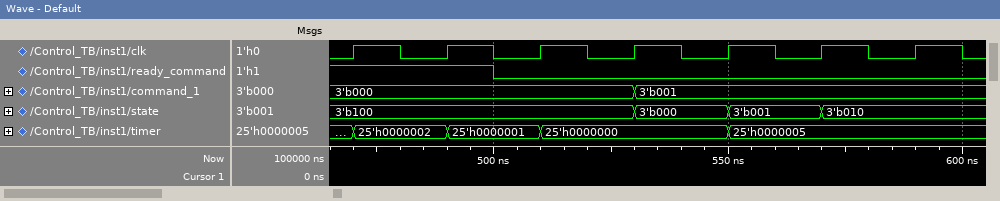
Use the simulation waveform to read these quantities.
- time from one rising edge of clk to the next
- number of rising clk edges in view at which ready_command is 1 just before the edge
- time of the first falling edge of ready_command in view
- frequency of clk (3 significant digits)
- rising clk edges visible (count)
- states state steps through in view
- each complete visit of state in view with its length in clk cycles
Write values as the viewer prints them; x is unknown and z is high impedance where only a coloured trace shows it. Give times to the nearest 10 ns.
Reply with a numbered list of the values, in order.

1. 20 ns
2. 2
3. 500 ns
4. 50.0 MHz
5. 7
6. 3'b100, 3'b000, 3'b001, 3'b010
7. 3'b000: 1, 3'b001: 1
